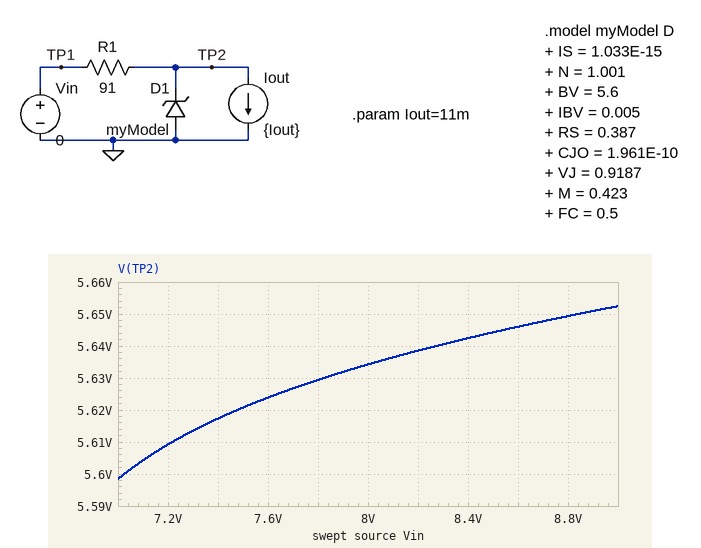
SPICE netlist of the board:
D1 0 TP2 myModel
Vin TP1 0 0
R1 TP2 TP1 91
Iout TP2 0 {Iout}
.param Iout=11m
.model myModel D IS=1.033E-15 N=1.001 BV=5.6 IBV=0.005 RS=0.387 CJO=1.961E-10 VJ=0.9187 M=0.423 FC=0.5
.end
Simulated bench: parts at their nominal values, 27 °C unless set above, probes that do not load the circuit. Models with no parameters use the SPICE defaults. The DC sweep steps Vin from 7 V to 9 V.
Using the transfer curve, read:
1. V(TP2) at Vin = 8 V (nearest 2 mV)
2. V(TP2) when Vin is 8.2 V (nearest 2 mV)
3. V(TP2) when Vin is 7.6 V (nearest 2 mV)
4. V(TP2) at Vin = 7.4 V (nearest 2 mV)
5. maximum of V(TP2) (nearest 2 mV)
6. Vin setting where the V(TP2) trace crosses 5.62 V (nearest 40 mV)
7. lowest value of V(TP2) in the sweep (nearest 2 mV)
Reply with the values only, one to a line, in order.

5.634 V
5.638 V
5.624 V
5.618 V
5.652 V
7.48 V
5.598 V
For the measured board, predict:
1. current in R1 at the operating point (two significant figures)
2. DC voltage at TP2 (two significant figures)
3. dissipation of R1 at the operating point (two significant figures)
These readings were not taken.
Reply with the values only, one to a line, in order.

8.2 mA
-740 mV
6.1 mW
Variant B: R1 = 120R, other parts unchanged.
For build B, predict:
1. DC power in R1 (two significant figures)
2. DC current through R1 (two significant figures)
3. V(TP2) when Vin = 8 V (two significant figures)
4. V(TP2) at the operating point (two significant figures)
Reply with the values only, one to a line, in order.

4.8 mW
6.3 mA
5.6 V
-760 mV
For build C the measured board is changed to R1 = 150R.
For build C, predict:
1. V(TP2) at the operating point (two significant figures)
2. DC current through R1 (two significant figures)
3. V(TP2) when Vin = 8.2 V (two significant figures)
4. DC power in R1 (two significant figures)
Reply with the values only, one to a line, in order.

-760 mV
5.1 mA
5.6 V
3.9 mW
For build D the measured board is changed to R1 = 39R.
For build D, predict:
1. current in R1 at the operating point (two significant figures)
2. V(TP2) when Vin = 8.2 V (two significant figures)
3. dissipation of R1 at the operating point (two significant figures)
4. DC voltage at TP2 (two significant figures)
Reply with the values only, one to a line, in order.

11 mA
5.7 V
4.7 mW
-430 mV
